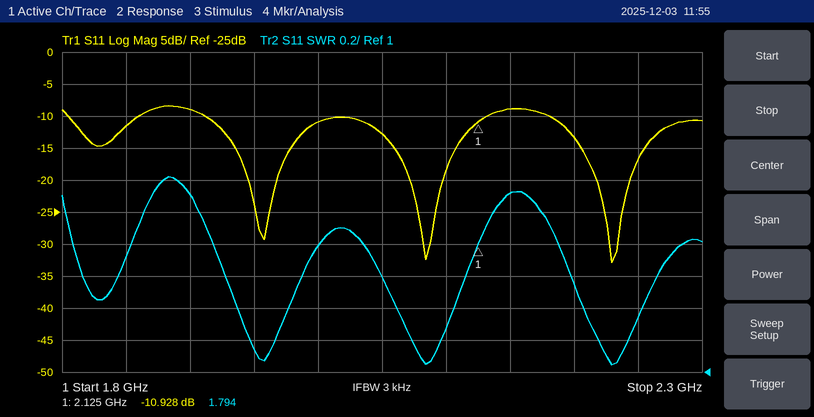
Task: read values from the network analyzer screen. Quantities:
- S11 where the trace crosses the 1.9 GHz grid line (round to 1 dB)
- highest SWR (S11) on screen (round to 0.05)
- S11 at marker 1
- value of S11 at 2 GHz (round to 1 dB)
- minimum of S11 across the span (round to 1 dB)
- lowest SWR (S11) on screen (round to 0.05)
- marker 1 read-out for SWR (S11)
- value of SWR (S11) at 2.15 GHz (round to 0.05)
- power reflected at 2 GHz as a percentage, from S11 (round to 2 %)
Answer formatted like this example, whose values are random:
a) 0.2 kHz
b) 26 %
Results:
a) -9 dB
b) 2.20
c) -10.928 dB
d) -11 dB
e) -33 dB
f) 1.05
g) 1.794
h) 2.10
i) 8 %
